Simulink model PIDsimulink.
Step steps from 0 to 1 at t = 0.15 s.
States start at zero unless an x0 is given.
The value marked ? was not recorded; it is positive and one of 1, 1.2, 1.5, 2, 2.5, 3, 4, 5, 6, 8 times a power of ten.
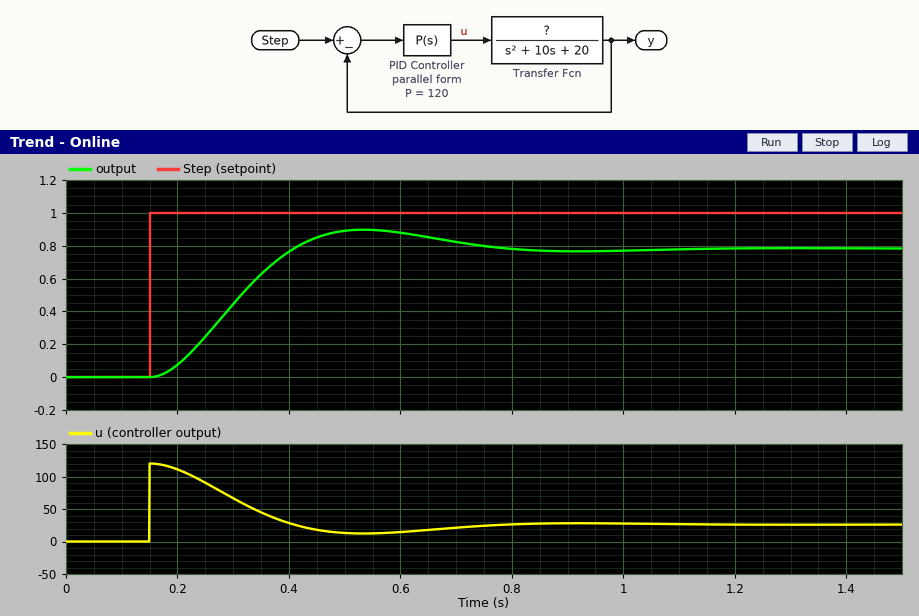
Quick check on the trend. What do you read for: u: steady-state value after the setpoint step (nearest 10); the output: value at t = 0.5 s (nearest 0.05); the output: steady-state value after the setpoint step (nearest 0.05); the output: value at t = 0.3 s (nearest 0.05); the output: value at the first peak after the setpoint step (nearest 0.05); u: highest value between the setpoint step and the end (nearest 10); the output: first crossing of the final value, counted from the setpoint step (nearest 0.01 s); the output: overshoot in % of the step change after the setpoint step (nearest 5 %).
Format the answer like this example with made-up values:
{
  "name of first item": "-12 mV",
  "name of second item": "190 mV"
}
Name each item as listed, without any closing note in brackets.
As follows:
{
  "u: steady-state value after the setpoint step": "30",
  "the output: value at t = 0.5 s": "0.90",
  "the output: steady-state value after the setpoint step": "0.80",
  "the output: value at t = 0.3 s": "0.45",
  "the output: value at the first peak after the setpoint step": "0.90",
  "u: highest value between the setpoint step and the end": "120",
  "the output: first crossing of the final value, counted from the setpoint step": "0.26 s",
  "the output: overshoot in % of the step change after the setpoint step": "15 %"
}
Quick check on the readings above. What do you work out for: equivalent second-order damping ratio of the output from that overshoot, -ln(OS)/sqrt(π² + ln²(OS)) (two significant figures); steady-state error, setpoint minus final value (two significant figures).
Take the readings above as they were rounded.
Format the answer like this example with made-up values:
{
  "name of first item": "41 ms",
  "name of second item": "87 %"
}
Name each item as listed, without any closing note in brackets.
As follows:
{
  "equivalent second-order damping ratio of the output from that overshoot, -ln(OS)/sqrt(π² + ln²(OS))": "0.52",
  "steady-state error, setpoint minus final value": "0.20"
}
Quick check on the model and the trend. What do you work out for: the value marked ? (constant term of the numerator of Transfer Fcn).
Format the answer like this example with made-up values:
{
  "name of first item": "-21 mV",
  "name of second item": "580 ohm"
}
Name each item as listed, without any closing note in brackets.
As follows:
{
  "the value marked ?": "0.6"
}
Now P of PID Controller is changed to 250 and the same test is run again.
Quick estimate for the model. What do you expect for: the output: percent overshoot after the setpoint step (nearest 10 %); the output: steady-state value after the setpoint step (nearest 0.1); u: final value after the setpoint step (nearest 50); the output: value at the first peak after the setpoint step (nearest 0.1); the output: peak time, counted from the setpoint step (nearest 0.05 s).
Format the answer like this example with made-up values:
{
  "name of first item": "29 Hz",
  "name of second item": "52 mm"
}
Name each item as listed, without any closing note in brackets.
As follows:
{
  "the output: percent overshoot after the setpoint step": "30 %",
  "the output: steady-state value after the setpoint step": "0.9",
  "u: final value after the setpoint step": "50",
  "the output: value at the first peak after the setpoint step": "1.1",
  "the output: peak time, counted from the setpoint step": "0.25 s"
}
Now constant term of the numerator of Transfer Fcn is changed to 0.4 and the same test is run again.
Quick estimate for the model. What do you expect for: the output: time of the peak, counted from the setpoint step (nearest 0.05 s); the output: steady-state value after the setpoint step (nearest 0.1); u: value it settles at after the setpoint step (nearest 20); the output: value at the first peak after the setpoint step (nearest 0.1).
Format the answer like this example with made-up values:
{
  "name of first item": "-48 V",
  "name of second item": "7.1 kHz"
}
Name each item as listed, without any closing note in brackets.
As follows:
{
  "the output: time of the peak, counted from the setpoint step": "0.50 s",
  "the output: steady-state value after the setpoint step": "0.7",
  "u: value it settles at after the setpoint step": "40",
  "the output: value at the first peak after the setpoint step": "0.8"
}
